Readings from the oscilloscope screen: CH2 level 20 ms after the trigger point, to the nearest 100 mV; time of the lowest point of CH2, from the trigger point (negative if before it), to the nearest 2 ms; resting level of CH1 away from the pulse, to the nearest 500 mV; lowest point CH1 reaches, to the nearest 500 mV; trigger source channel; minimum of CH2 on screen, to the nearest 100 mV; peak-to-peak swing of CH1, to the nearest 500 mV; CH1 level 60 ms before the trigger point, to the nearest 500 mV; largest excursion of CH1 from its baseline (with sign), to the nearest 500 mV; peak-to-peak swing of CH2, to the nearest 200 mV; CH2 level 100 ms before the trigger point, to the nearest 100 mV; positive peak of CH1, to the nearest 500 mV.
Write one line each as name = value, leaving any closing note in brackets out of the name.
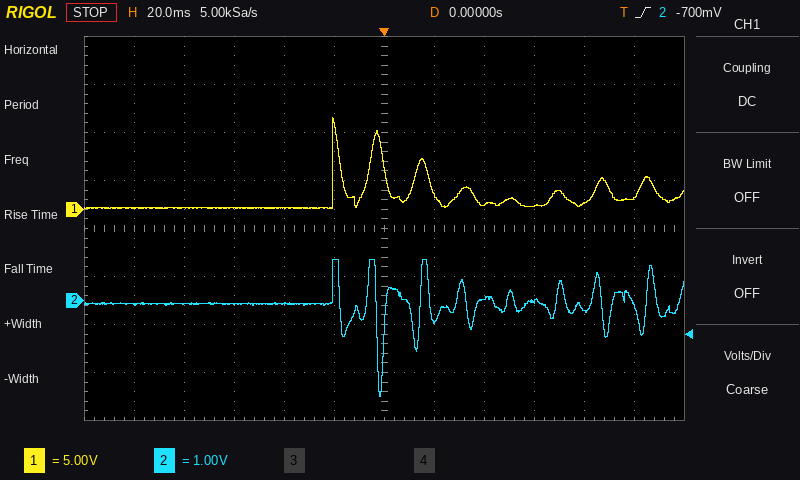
CH2 level 20 ms after the trigger point, to the nearest 100 mV = -400 mV
time of the lowest point of CH2, from the trigger point (negative if before it), to the nearest 2 ms = -2 ms
resting level of CH1 away from the pulse, to the nearest 500 mV = 0.0 V
lowest point CH1 reaches, to the nearest 500 mV = 0.0 V
trigger source channel = CH2
minimum of CH2 on screen, to the nearest 100 mV = -2.0 V
peak-to-peak swing of CH1, to the nearest 500 mV = 9.5 V
CH1 level 60 ms before the trigger point, to the nearest 500 mV = 0.0 V
largest excursion of CH1 from its baseline (with sign), to the nearest 500 mV = +9.5 V
peak-to-peak swing of CH2, to the nearest 200 mV = 2.8 V
CH2 level 100 ms before the trigger point, to the nearest 100 mV = -100 mV
positive peak of CH1, to the nearest 500 mV = 9.5 V
